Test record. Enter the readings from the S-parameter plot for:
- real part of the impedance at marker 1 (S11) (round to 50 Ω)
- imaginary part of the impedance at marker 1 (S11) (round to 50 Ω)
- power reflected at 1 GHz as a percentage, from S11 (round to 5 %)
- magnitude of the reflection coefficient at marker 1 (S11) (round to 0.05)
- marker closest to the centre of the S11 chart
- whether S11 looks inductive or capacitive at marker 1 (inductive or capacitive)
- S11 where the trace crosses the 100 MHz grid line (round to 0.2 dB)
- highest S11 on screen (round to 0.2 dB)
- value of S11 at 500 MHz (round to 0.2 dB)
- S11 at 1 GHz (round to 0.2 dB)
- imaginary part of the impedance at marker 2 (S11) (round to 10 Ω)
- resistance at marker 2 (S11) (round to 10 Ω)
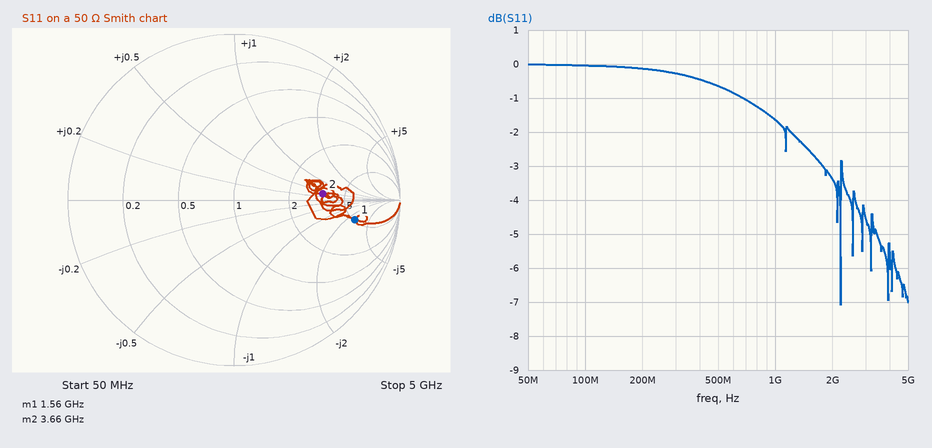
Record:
250 Ω
-150 Ω
70 %
0.75
marker 2
capacitive
0.0 dB
0.0 dB
-0.6 dB
-1.6 dB
+20 Ω
160 Ω
